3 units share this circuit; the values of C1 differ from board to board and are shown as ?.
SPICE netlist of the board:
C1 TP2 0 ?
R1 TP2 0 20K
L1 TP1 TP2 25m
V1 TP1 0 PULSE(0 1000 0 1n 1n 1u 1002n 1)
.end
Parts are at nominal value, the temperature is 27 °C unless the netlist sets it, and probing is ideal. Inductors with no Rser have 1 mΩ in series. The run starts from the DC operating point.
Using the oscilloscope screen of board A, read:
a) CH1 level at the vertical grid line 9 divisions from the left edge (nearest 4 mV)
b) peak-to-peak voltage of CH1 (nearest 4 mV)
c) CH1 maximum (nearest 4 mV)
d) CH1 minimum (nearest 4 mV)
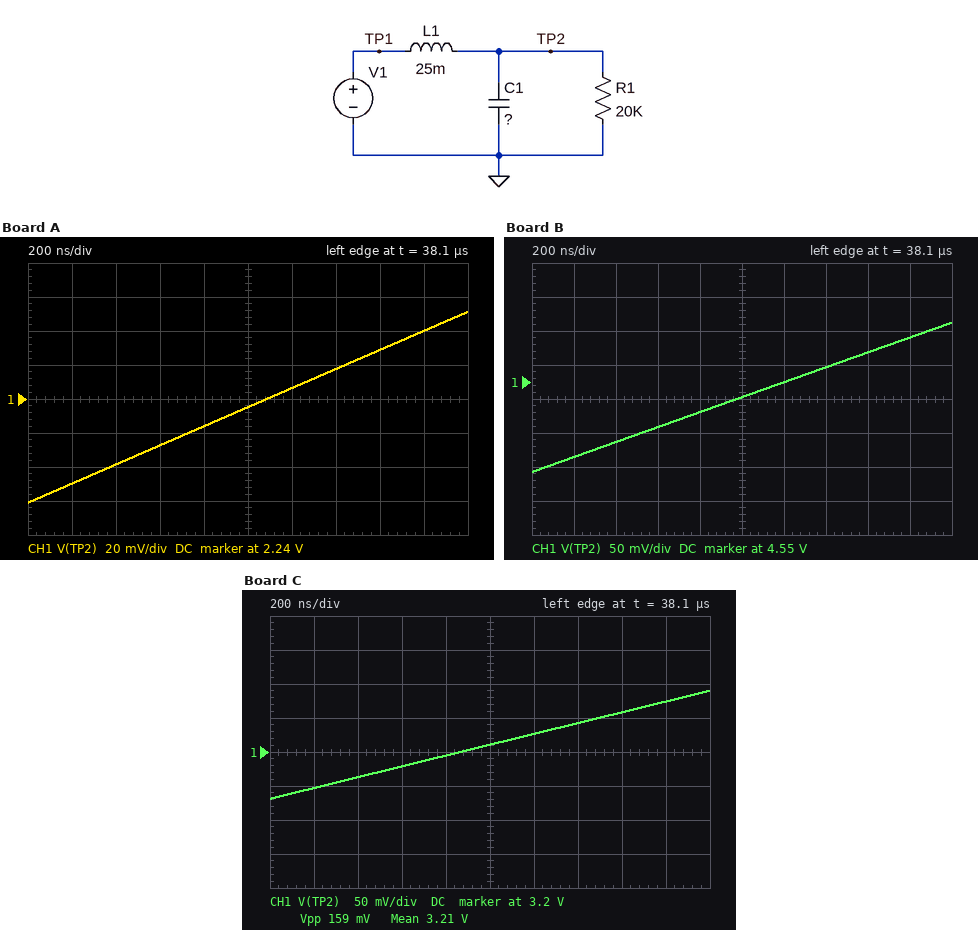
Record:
2.280 V
112 mV
2.292 V
2.180 V
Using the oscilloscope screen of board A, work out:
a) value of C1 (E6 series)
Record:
680 nF
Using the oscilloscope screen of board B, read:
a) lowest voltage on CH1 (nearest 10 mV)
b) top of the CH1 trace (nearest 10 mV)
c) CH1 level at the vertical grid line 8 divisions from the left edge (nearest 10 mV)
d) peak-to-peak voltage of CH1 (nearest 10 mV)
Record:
4.42 V
4.64 V
4.59 V
220 mV
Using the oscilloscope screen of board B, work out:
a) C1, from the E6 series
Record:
330 nF
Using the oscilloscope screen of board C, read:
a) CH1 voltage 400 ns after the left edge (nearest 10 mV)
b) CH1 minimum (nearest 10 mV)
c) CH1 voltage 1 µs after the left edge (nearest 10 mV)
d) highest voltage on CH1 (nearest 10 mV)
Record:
3.16 V
3.13 V
3.21 V
3.29 V
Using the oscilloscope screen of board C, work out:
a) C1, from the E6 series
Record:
470 nF
